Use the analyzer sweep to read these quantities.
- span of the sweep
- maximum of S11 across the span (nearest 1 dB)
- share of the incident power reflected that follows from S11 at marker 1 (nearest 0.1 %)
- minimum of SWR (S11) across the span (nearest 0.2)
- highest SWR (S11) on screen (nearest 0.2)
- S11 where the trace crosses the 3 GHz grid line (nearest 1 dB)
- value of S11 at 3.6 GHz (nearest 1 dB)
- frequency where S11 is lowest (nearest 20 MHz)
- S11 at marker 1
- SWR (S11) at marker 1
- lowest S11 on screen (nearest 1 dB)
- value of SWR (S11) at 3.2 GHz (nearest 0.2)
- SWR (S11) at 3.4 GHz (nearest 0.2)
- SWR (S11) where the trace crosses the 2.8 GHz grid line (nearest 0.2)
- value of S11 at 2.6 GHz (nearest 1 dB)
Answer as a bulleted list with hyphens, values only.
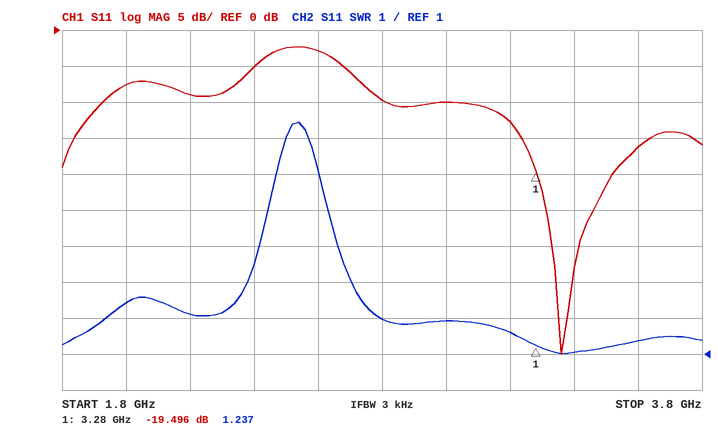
- 2 GHz
- -2 dB
- 1.1 %
- 1.0
- 7.4
- -10 dB
- -16 dB
- 3.36 GHz
- -19.496 dB
- 1.237
- -45 dB
- 1.6
- 1.0
- 2.0
- -3 dB
